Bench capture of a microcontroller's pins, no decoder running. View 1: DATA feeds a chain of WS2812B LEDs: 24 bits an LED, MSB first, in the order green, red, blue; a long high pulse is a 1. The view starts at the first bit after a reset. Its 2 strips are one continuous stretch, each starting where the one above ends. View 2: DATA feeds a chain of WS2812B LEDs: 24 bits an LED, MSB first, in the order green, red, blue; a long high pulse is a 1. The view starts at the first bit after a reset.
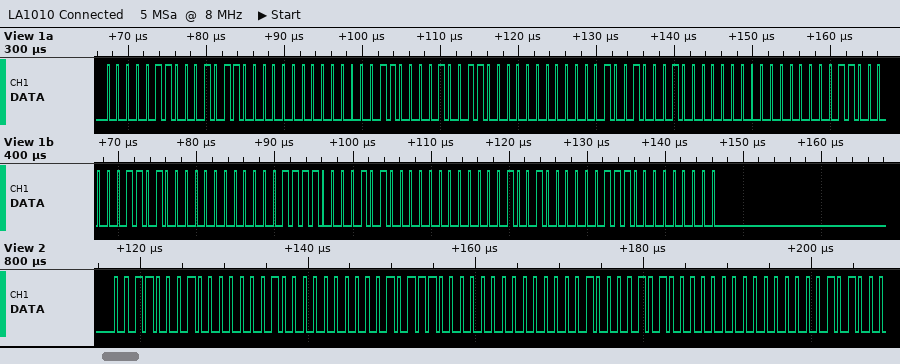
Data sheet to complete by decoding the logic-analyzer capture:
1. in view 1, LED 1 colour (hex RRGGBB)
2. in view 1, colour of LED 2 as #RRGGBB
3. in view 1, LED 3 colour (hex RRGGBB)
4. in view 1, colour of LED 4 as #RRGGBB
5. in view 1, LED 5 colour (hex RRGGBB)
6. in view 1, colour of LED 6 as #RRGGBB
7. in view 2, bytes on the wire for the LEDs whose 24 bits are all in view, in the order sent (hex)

#2C0600
#260C00
#201200
#1A1800
#141E00
#0E2400
31 01 00 2E 00 04 28 00 0A
